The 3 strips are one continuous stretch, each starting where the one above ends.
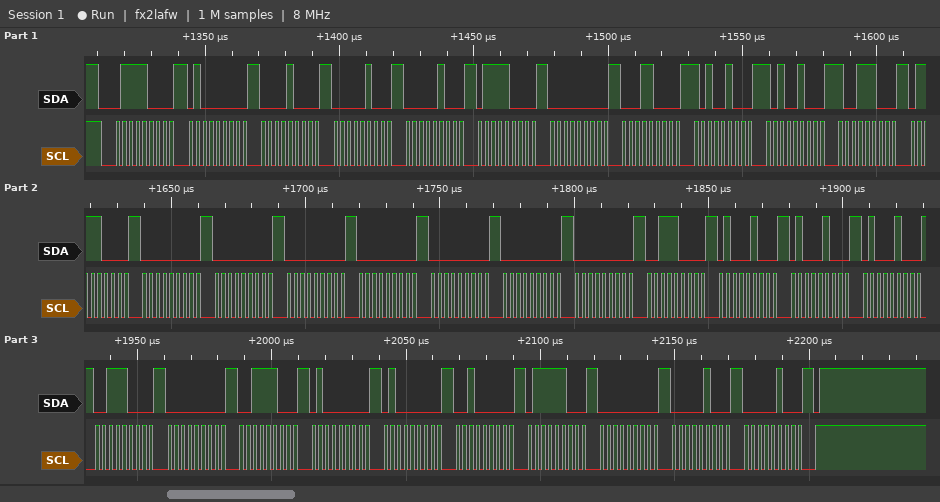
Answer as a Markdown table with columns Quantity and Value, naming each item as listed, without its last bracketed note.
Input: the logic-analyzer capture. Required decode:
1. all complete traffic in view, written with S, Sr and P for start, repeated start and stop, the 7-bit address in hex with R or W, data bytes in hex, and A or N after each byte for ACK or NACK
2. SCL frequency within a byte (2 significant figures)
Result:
| Quantity | Value |
|---|---|
| all complete traffic in view, written with S, Sr and P for start, repeated start and stop, the 7-bit address in hex with R or W, data bytes in hex, and A or N after each byte for ACK or NACK | S 3CW A 40 A 08 A 04 A 04 A 78 A 00 A 18 A A4 A A4 A 9C A 78 A 00 A 00 A 00 A 00 A 00 A 00 A 00 A 38 A 44 A 44 A 44 A 38 A 00 A 3C A 40 A 40 A 20 A 7C A 00 A 04 A 04 A P |
| SCL frequency within a byte | 400 kHz |
